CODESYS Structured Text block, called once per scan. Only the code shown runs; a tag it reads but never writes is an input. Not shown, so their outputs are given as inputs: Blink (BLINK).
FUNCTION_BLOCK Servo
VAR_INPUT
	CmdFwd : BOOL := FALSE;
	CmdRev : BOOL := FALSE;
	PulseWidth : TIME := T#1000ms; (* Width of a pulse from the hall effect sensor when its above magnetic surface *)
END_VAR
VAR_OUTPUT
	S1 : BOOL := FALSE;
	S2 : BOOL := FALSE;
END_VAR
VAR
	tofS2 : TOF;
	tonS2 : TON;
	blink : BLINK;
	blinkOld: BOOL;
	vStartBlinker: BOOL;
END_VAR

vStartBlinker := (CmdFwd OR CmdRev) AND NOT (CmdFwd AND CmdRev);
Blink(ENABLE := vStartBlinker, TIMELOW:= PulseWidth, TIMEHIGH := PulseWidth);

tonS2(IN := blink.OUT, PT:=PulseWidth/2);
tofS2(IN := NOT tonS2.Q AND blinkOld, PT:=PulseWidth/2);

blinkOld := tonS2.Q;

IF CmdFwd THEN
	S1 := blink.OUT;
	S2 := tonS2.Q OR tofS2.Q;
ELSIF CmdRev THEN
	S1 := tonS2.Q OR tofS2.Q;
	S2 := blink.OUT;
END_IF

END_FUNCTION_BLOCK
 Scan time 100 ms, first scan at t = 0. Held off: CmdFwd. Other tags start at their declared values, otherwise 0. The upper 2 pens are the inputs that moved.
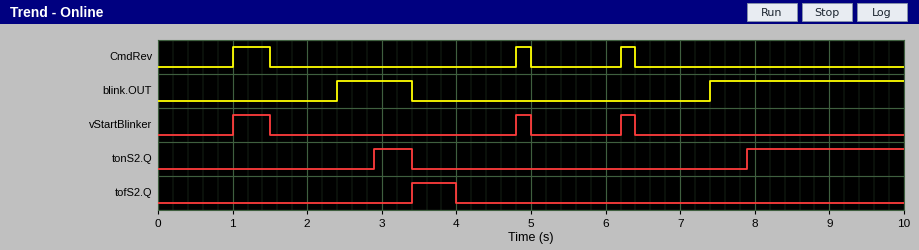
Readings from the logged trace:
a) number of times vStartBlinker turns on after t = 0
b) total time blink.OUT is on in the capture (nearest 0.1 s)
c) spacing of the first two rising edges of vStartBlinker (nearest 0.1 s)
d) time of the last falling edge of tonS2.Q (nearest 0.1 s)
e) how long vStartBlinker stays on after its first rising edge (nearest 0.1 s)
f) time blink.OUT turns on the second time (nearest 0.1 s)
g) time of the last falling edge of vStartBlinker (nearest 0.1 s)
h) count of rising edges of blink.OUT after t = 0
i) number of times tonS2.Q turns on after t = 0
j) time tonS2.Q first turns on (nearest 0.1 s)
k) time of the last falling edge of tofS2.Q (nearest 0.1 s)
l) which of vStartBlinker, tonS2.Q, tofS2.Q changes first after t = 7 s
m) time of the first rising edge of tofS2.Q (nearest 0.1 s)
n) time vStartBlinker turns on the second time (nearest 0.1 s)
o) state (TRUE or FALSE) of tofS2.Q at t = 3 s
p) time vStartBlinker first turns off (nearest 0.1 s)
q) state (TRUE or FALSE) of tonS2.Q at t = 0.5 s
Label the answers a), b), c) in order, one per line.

a) 3
b) 3.6 s
c) 3.8 s
d) 3.4 s
e) 0.5 s
f) 7.4 s
g) 6.4 s
h) 2
i) 2
j) 2.9 s
k) 4.0 s
l) tonS2.Q
m) 3.4 s
n) 4.8 s
o) FALSE
p) 1.5 s
q) FALSE
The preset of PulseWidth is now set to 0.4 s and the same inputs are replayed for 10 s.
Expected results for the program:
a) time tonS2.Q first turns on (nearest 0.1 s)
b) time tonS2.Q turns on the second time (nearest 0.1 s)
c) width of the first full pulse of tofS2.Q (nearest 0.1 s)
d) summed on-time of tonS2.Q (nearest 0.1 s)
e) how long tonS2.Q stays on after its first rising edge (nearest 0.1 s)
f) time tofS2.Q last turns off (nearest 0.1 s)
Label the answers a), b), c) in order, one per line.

a) 2.6 s
b) 7.6 s
c) 0.3 s
d) 3.2 s
e) 0.8 s
f) 3.7 s
